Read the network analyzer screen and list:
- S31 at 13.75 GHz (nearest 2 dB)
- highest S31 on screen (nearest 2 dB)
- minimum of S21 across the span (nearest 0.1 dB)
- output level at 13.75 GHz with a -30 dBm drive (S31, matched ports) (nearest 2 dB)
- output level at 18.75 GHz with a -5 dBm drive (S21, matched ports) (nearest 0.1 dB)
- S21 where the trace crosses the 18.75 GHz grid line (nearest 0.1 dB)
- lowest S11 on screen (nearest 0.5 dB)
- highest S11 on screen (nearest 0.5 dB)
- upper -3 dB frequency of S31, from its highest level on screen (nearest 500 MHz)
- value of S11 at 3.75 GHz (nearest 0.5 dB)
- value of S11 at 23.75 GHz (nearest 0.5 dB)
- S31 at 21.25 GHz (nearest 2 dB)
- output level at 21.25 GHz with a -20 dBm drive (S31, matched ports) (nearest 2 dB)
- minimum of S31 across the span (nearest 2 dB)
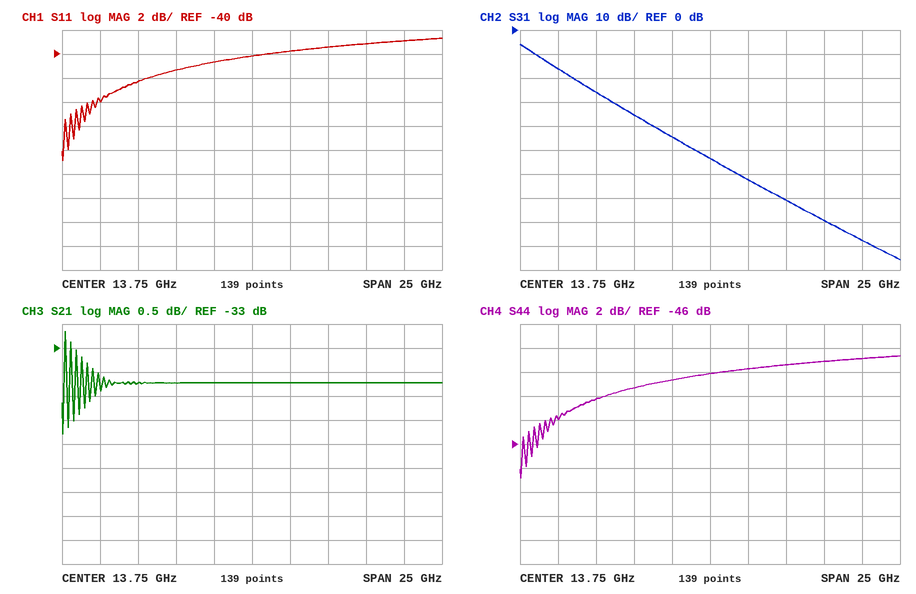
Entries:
-54 dB
-6 dB
-34.8 dB
-84 dBm
-38.7 dBm
-33.7 dB
-49.0 dB
-38.5 dB
2.0 GHz
-44.0 dB
-39.0 dB
-80 dB
-100 dBm
-96 dB
